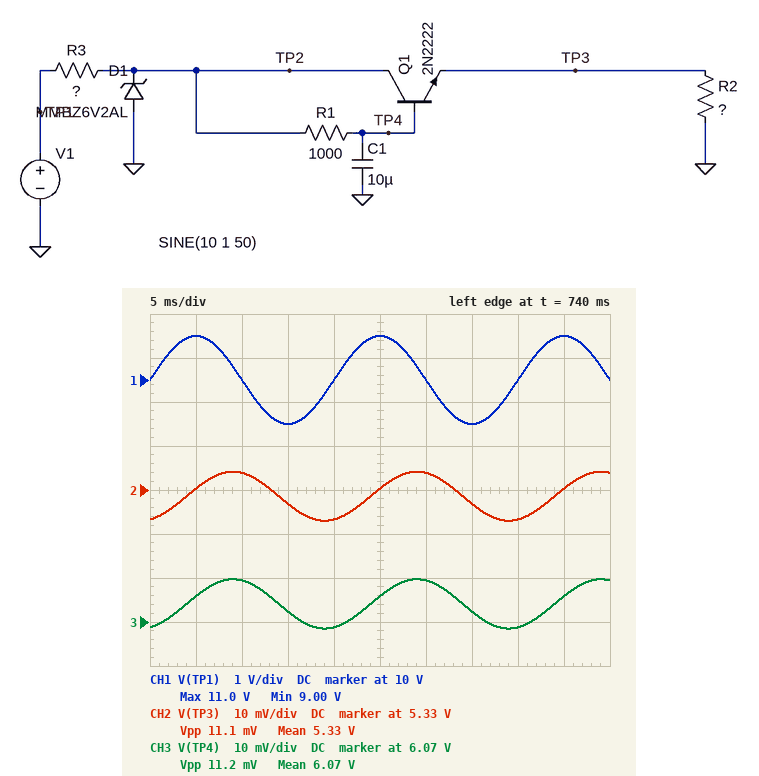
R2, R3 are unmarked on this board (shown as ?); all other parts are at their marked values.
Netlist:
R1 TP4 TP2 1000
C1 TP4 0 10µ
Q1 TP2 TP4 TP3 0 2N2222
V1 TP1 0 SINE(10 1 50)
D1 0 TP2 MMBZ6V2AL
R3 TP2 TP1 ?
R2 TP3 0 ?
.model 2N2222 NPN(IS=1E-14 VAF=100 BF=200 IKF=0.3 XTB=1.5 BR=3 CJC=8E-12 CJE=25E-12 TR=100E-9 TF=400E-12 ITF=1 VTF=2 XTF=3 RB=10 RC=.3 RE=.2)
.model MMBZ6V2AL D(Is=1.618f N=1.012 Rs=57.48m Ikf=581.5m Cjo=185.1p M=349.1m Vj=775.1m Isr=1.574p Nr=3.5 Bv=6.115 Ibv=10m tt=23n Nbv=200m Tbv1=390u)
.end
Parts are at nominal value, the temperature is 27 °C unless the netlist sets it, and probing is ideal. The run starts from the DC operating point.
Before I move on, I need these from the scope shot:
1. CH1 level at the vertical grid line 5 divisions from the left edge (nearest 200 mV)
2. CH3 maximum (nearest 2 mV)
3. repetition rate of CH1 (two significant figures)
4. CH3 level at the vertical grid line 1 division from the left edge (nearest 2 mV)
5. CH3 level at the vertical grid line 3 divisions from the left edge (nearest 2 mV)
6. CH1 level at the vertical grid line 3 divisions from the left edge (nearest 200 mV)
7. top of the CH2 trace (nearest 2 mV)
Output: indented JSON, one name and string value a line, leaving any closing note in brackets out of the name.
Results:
{
  "CH1 level at the vertical grid line 5 divisions from the left edge": "11.0 V",
  "CH3 maximum": "6.080 V",
  "repetition rate of CH1": "50 Hz",
  "CH3 level at the vertical grid line 1 division from the left edge": "6.076 V",
  "CH3 level at the vertical grid line 3 divisions from the left edge": "6.072 V",
  "CH1 level at the vertical grid line 3 divisions from the left edge": "9.0 V",
  "top of the CH2 trace": "5.334 V"
}
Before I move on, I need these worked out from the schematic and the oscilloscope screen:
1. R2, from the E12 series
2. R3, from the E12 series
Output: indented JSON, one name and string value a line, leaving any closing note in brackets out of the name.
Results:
{
  "R2, from the E12 series": "220 Ω",
  "R3, from the E12 series": "3.3 Ω"
}
